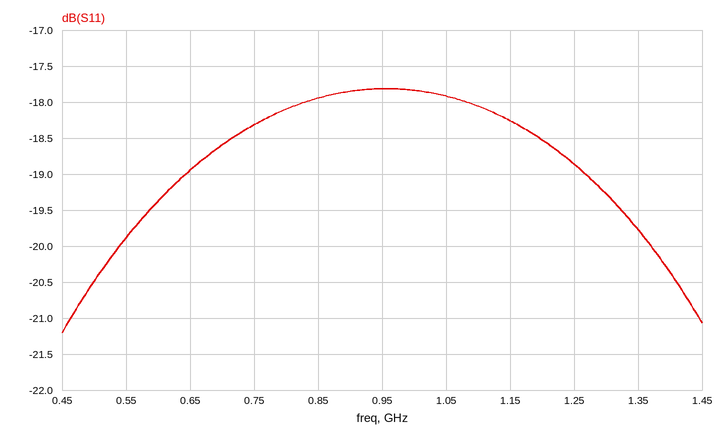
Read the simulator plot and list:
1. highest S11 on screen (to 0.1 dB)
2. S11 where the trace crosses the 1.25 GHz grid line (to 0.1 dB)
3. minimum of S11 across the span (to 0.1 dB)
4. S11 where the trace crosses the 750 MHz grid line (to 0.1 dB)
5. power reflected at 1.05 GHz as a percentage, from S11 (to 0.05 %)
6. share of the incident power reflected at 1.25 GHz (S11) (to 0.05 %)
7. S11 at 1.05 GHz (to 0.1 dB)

-17.8 dB
-18.9 dB
-21.2 dB
-18.3 dB
1.60 %
1.30 %
-17.9 dB
